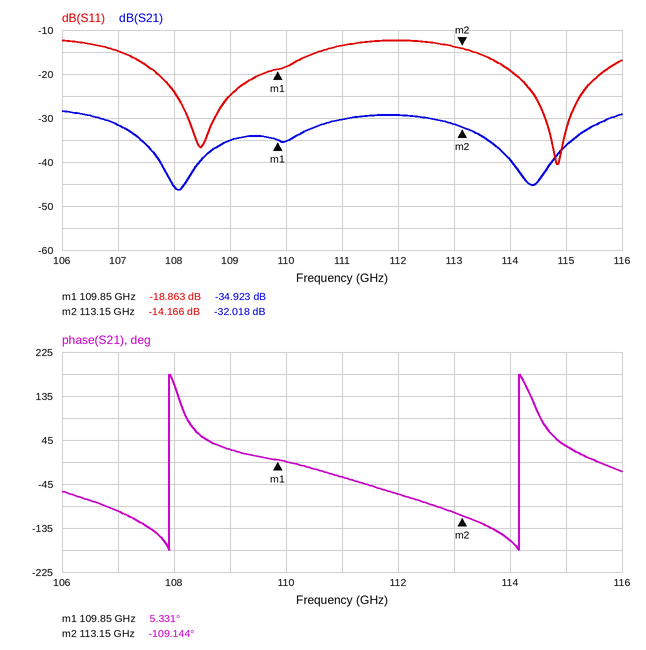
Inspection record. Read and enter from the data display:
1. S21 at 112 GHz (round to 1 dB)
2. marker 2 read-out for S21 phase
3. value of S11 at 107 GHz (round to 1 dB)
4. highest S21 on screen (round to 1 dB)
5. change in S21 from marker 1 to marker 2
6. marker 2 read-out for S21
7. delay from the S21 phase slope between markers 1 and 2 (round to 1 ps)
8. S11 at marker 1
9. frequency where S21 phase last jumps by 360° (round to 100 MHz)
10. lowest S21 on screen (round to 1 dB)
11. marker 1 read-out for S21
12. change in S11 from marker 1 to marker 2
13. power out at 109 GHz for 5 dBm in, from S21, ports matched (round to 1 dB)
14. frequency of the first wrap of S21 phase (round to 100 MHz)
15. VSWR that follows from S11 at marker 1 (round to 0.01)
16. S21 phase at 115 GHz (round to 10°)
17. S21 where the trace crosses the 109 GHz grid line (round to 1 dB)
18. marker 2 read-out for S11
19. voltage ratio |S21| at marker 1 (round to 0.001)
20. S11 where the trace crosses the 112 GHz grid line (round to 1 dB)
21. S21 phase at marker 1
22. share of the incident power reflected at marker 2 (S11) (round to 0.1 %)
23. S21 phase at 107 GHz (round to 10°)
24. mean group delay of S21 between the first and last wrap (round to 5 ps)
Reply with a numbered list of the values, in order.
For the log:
1. -29 dB
2. -109.144°
3. -15 dB
4. -28 dB
5. 2.905 dB
6. -32.018 dB
7. 96 ps
8. -18.863 dB
9. 114.2 GHz
10. -46 dB
11. -34.923 dB
12. 4.697 dB
13. -30 dBm
14. 107.9 GHz
15. 1.26
16. 30°
17. -35 dB
18. -14.166 dB
19. 0.018
20. -12 dB
21. 5.331°
22. 3.8 %
23. -100°
24. 160 ps
